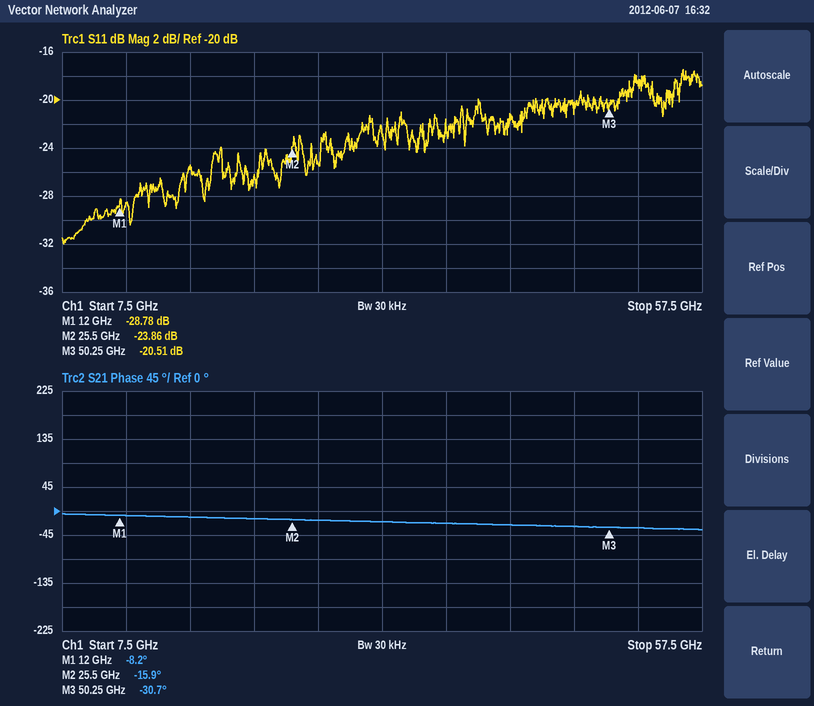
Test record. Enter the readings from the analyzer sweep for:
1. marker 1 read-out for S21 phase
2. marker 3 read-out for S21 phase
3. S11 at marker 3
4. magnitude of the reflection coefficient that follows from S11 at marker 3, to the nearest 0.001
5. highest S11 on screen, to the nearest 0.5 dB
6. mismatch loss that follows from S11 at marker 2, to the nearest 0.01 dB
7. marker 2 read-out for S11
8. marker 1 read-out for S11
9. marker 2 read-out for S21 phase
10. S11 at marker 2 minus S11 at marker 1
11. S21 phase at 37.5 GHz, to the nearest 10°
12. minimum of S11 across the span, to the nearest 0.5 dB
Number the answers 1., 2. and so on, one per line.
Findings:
1. -8.2°
2. -30.7°
3. -20.51 dB
4. 0.094
5. -17.5 dB
6. 0.02 dB
7. -23.86 dB
8. -28.78 dB
9. -15.9°
10. 4.92 dB
11. -20°
12. -32.0 dB
